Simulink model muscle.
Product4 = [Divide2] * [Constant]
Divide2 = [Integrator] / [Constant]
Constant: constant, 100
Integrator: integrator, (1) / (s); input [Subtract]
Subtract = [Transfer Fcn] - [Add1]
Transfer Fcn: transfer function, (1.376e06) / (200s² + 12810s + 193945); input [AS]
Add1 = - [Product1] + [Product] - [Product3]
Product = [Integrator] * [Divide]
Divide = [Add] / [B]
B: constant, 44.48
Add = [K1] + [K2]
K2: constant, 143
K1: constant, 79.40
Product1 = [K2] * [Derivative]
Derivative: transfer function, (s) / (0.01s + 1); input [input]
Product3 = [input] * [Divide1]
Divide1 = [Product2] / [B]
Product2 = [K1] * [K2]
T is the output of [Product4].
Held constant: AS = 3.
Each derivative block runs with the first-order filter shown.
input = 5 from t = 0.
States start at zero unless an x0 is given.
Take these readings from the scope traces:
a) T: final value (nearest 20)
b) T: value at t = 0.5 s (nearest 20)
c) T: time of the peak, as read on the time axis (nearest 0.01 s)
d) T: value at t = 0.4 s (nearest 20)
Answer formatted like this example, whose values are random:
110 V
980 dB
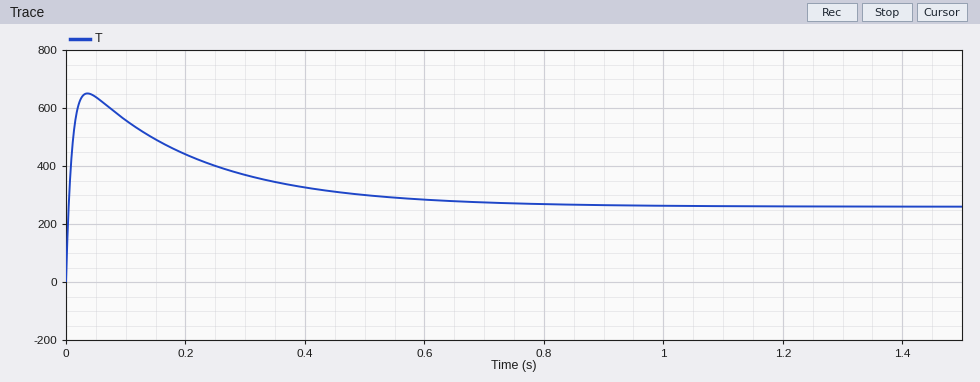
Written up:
260
300
0.04 s
320
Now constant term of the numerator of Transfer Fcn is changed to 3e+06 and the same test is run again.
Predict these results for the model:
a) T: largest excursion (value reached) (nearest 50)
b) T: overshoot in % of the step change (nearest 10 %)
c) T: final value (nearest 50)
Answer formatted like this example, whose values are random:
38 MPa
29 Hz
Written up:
650
150 %
250
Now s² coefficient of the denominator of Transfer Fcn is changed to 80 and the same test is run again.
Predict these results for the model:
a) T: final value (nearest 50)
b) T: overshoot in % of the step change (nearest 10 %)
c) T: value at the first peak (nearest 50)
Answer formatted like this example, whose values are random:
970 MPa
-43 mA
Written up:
250
150 %
650
